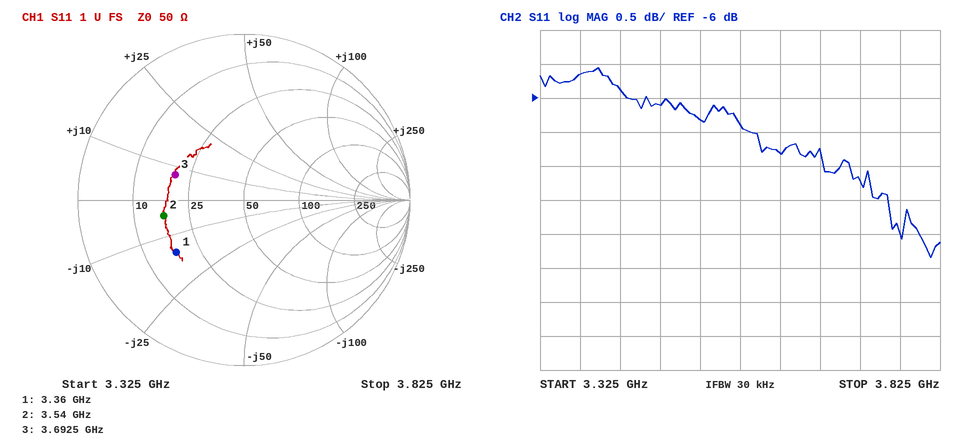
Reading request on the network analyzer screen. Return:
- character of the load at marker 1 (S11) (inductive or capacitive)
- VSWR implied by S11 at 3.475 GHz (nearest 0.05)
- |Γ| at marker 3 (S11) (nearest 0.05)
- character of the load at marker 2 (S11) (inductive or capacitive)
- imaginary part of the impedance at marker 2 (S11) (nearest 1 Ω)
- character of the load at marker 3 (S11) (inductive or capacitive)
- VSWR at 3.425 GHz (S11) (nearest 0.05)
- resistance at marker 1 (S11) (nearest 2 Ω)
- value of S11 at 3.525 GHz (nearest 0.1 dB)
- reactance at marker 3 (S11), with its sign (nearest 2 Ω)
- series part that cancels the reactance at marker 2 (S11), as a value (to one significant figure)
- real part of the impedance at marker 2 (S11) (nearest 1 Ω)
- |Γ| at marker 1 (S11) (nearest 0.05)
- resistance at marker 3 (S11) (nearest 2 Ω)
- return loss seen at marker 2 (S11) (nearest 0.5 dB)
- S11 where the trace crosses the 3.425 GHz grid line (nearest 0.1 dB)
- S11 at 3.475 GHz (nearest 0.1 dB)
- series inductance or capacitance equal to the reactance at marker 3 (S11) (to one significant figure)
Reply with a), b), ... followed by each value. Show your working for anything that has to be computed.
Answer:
a) capacitive
b) |Γ| = 10^(-6.1/20) = 0.4955; VSWR = (1 + 0.4955)/(1 − 0.4955) ≈ 2.96, so 2.95 to the nearest 0.05
c) 0.45
d) capacitive
e) -4 Ω
f) inductive
g) |Γ| = 10^(-5.9/20) = 0.5070; VSWR = (1 + 0.5070)/(1 − 0.5070) ≈ 3.06, so 3.05 to the nearest 0.05
h) 18 Ω
i) -6.3 dB
j) +8 Ω
k) L = 4 Ω/(2π × 3.54 GHz) ≈ 180 pH, so 200 pH to one significant figure
l) 17 Ω
m) 0.50
n) 20 Ω
o) 6.0 dB
p) -5.9 dB
q) -6.1 dB
r) L = 8 Ω/(2π × 3.6925 GHz) ≈ 345 pH, so 300 pH to one significant figure
